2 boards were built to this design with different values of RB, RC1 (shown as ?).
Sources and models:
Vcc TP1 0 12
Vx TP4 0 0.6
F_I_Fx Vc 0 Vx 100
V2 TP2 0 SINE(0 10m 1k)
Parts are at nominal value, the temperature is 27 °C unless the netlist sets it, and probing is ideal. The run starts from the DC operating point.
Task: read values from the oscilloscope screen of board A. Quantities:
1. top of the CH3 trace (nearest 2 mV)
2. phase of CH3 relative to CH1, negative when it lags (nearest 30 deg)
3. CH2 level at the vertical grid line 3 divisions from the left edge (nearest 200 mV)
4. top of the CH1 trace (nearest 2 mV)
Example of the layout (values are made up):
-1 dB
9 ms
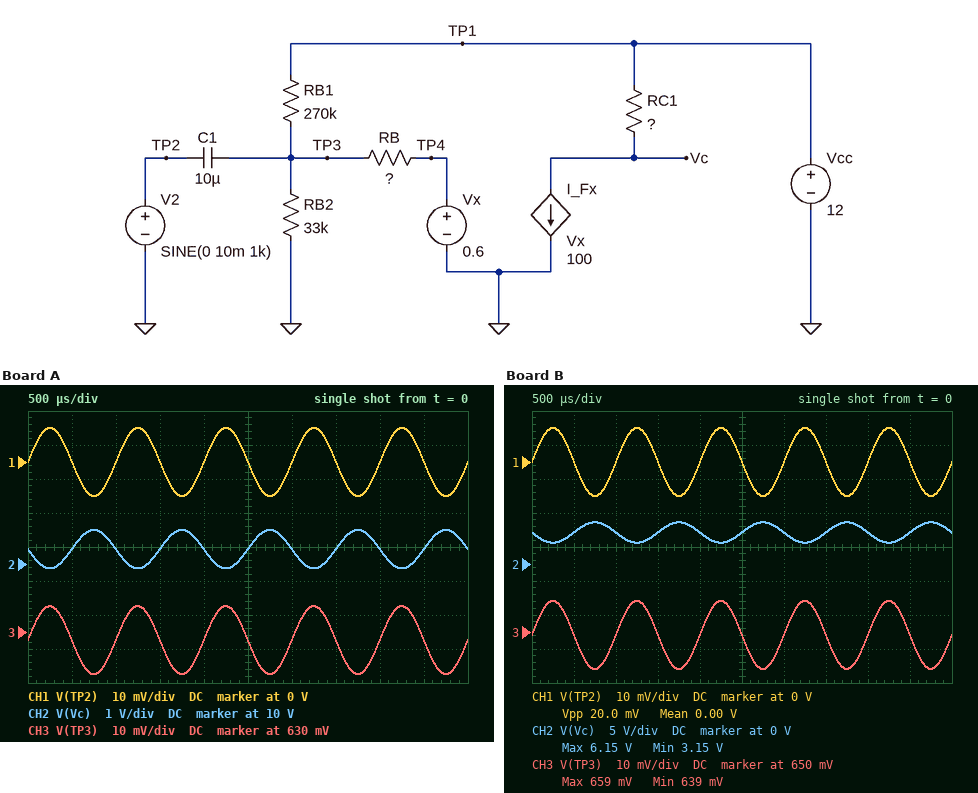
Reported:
638 mV
0 deg
10.4 V
10 mV
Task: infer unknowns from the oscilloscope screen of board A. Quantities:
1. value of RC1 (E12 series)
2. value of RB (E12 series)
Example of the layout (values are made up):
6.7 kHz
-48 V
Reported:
680 Ω
1.2 kΩ
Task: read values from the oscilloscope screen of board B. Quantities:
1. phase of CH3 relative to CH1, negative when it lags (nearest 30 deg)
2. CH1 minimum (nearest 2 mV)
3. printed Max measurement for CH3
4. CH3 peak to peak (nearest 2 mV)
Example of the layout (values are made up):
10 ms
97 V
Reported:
0 deg
-10 mV
659 mV
20 mV
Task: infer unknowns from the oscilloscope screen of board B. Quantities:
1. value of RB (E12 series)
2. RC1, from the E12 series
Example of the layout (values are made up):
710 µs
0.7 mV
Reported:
2.2 kΩ
3.3 kΩ
